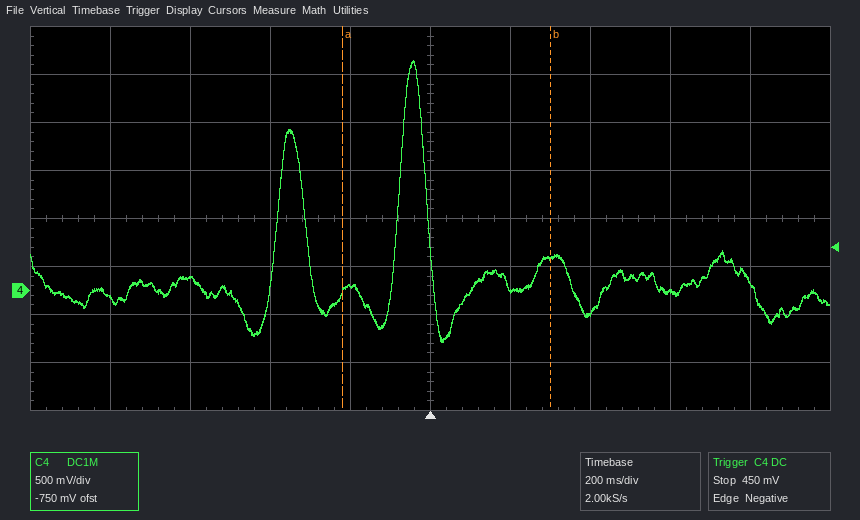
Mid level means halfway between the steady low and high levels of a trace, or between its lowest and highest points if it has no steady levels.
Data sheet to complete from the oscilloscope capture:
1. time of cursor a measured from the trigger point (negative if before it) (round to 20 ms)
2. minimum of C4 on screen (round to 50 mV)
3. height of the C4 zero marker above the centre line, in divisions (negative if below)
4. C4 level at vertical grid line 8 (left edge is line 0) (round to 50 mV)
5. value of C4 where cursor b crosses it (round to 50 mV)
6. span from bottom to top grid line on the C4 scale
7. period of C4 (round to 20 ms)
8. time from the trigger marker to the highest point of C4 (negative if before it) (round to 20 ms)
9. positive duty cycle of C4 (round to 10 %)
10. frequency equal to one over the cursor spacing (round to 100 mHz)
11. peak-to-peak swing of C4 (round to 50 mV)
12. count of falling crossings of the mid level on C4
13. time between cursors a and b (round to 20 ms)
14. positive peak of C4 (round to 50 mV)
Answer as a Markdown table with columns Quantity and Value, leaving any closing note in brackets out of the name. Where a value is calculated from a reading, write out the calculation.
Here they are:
| Quantity | Value |
|---|---|
| time of cursor a measured from the trigger point (negative if before it) | -220 ms |
| minimum of C4 on screen | -550 mV |
| height of the C4 zero marker above the centre line, in divisions | -1.5 div |
| C4 level at vertical grid line 8 (left edge is line 0) | 0 mV |
| value of C4 where cursor b crosses it | 350 mV |
| span from bottom to top grid line on the C4 scale | 4 V |
| period of C4 | 300 ms |
| time from the trigger marker to the highest point of C4 (negative if before it) | -40 ms |
| positive duty cycle of C4 | 20 % |
| frequency equal to one over the cursor spacing | 1 / 520 ms ≈ 1.9 Hz |
| peak-to-peak swing of C4 | 2.40 V − (-550 mV) = 2.95 V |
| count of falling crossings of the mid level on C4 | 2 |
| time between cursors a and b | 520 ms |
| positive peak of C4 | 2.40 V |
